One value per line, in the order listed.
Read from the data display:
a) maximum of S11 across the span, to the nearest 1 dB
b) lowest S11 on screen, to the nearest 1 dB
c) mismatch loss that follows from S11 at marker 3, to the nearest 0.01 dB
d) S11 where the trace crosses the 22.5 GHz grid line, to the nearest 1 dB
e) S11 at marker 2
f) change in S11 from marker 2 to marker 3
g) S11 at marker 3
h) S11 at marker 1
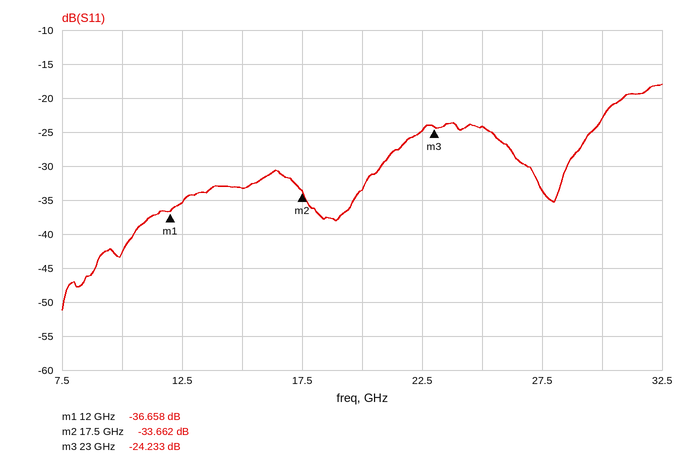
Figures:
-18 dB
-51 dB
0.02 dB
-25 dB
-33.662 dB
9.429 dB
-24.233 dB
-36.658 dB
